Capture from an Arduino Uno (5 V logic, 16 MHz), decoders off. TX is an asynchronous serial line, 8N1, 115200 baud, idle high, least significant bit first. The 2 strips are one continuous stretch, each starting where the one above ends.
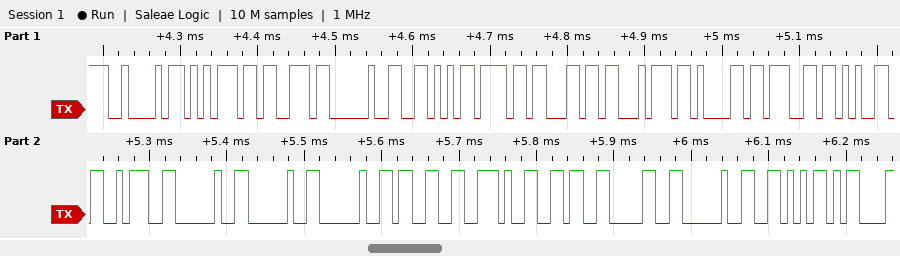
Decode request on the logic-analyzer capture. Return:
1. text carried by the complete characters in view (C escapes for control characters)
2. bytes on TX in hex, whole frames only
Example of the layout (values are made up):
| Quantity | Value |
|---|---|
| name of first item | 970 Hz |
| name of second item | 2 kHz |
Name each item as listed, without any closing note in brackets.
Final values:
| Quantity | Value |
|---|---|
| text carried by the complete characters in view | "Bus Voltage:   3.60 V\r" |
| bytes on TX in hex, whole frames only | 42 75 73 20 56 6F 6C 74 61 67 65 3A 20 20 20 33 2E 36 30 20 56 0D |
